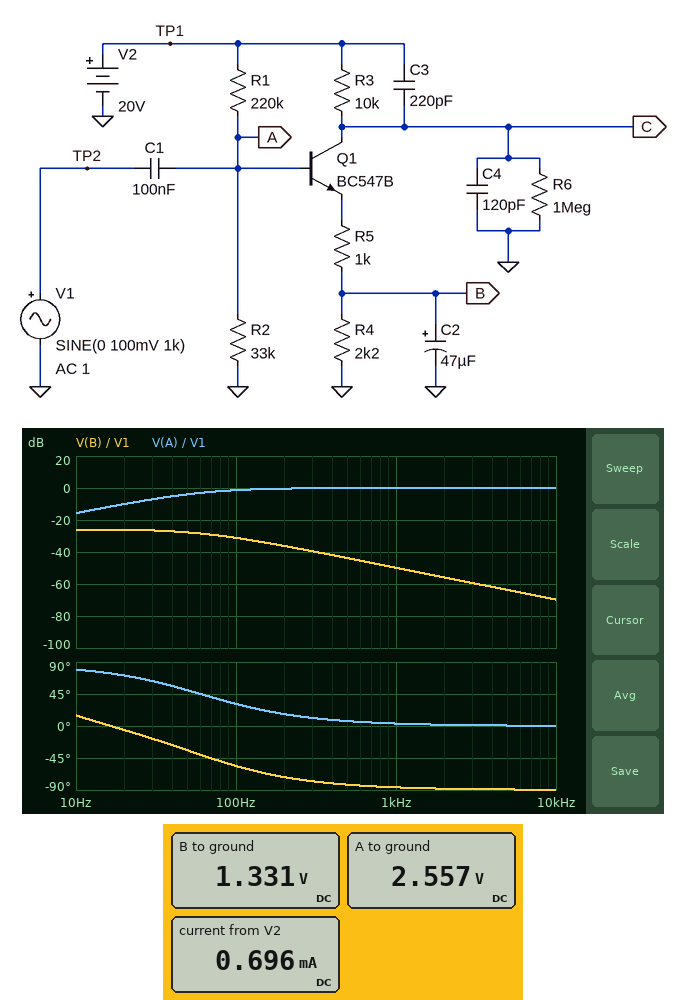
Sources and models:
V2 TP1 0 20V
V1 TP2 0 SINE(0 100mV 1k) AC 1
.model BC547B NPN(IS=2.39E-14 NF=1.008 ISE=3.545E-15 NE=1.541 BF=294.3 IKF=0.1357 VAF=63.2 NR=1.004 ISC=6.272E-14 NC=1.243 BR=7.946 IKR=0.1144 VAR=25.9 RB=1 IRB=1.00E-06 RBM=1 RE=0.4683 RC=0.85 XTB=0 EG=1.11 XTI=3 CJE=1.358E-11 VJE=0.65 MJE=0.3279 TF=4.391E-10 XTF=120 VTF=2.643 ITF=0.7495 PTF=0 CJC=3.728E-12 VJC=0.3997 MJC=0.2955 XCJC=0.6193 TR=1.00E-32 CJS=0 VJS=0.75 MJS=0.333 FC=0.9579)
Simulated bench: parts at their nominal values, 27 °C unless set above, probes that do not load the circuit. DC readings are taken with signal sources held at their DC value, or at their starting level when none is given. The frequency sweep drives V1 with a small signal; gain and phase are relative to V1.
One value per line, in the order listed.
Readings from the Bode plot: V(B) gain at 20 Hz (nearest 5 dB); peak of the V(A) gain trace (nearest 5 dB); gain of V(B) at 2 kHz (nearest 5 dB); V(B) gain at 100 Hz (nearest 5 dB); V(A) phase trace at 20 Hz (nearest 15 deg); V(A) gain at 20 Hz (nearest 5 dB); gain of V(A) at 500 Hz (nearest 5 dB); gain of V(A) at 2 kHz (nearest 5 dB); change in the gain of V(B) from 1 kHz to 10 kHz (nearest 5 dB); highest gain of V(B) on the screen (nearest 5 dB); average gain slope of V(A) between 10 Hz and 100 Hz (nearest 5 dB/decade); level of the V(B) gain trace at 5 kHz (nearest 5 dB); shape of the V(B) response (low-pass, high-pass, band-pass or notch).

-25 dB
0 dB
-55 dB
-30 dB
75 deg
-10 dB
0 dB
0 dB
-20 dB
-25 dB
15 dB/decade
-65 dB
low-pass
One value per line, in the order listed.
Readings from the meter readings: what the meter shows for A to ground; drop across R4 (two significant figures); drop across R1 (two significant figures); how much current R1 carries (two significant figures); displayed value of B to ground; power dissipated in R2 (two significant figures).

2.557 V
1.3 V
17 V
79 µA
1.331 V
200 µW
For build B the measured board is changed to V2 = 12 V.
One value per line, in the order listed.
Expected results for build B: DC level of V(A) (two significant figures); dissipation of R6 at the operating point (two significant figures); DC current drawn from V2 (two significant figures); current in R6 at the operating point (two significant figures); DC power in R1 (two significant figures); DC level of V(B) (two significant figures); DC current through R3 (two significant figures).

1.5 V
81 µW
350 µA
9.0 µA
500 µW
640 mV
300 µA
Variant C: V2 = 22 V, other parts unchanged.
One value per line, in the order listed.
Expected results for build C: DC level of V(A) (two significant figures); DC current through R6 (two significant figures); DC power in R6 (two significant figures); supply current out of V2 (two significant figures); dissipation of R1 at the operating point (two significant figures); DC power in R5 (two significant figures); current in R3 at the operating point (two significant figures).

2.8 V
15 µA
230 µW
780 µA
1.7 mW
470 µW
700 µA
